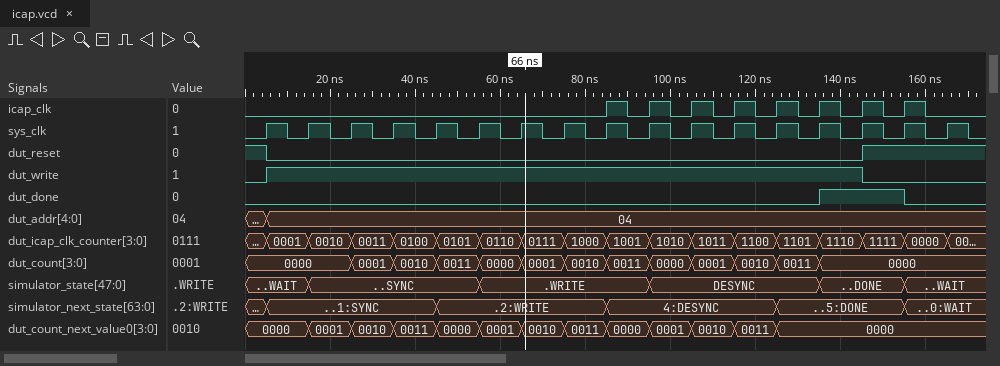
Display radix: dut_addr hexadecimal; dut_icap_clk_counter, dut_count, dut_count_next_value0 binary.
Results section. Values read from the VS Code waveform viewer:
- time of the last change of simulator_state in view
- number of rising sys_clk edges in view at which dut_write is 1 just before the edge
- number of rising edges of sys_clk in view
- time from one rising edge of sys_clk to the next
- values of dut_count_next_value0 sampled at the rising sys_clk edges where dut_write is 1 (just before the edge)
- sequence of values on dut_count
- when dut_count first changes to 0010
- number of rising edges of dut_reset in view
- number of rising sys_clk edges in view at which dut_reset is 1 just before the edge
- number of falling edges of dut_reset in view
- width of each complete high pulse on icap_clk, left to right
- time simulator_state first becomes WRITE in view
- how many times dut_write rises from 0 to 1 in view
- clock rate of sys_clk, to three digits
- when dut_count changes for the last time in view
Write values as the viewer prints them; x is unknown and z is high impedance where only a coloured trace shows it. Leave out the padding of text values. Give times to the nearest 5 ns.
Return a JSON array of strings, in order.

["155 ns", "14", "17", "10 ns", "0000, 0001, 0010, 0011, 0000, 0001, 0010, 0011, 0000, 0001, 0010, 0011, 0000, 0000", "0000, 0001, 0010, 0011, 0000, 0001, 0010, 0011, 0000, 0001, 0010, 0011, 0000", "35 ns", "1", "3", "1", "5 ns, 5 ns, 5 ns, 5 ns, 5 ns, 5 ns, 5 ns, 5 ns", "55 ns", "1", "100 MHz", "135 ns"]
